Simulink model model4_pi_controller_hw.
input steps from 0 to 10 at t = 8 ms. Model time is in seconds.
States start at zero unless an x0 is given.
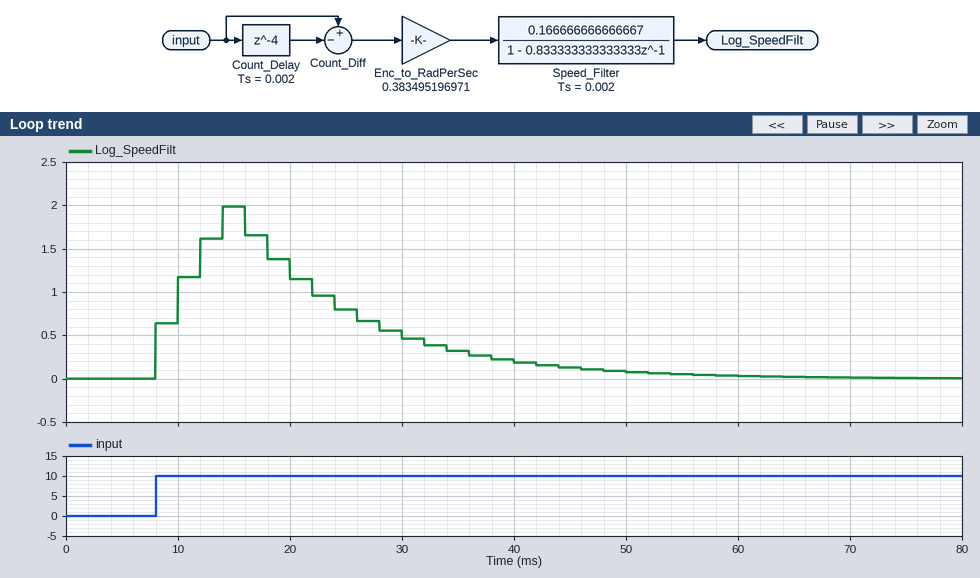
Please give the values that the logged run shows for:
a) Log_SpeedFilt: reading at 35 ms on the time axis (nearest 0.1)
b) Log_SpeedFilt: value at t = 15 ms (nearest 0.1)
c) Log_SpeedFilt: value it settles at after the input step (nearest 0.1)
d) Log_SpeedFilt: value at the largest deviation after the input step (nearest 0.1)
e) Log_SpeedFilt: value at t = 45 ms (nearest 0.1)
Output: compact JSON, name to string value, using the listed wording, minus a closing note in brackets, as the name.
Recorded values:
{"Log_SpeedFilt: reading at 35 ms on the time axis": "0.3", "Log_SpeedFilt: value at t = 15 ms": "2.0", "Log_SpeedFilt: value it settles at after the input step": "0.0", "Log_SpeedFilt: value at the largest deviation after the input step": "2.0", "Log_SpeedFilt: value at t = 45 ms": "0.1"}
